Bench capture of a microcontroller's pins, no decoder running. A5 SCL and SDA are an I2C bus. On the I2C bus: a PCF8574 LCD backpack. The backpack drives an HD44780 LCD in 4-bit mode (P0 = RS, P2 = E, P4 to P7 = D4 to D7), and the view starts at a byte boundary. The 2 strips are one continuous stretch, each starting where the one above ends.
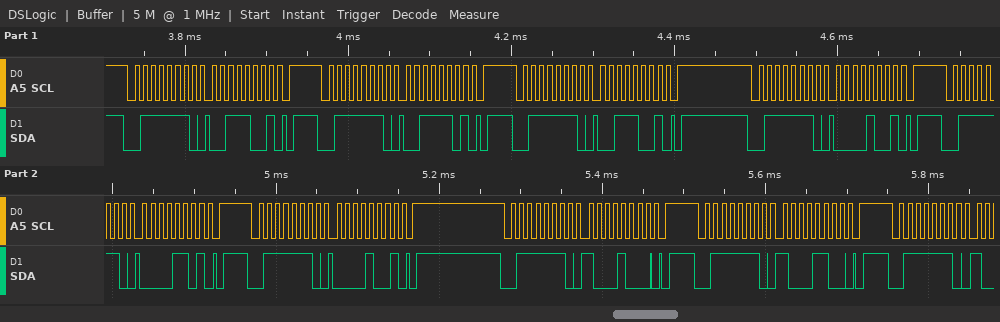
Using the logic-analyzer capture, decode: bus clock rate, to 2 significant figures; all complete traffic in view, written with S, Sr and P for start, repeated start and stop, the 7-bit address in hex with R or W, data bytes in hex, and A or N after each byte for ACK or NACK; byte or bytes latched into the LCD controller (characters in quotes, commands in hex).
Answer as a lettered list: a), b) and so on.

a) 100 kHz
b) S 3FW A 39 A P S 3FW A 3D A P S 3FW A 39 A P S 3FW A 09 A P S 3FW A 0D A P S 3FW A 09 A P S 3FW A 88 A P S 3FW A 8C A P S 3FW A
c) '0'
